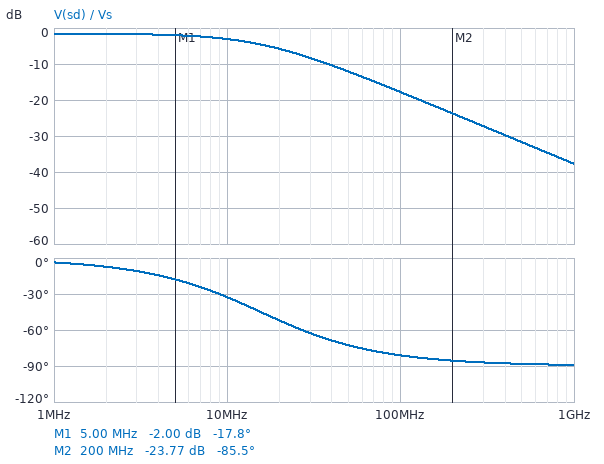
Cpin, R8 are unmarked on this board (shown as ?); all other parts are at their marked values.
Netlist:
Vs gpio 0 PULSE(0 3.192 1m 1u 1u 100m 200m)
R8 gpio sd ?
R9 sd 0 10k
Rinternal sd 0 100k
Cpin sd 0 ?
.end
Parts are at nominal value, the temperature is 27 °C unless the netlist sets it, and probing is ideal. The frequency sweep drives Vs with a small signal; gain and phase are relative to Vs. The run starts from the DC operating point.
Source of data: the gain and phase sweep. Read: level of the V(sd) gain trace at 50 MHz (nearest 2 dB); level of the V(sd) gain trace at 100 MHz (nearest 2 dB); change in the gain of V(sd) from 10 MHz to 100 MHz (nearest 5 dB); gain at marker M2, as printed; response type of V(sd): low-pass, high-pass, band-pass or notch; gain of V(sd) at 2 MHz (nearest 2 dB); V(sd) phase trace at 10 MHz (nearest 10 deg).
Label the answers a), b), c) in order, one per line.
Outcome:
a) -12 dB
b) -18 dB
c) -15 dB
d) -23.77 dB
e) low-pass
f) -2 dB
g) -30 deg
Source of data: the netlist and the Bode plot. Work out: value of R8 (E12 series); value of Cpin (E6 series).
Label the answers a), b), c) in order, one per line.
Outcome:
a) 1.8 kΩ
b) 6.8 pF
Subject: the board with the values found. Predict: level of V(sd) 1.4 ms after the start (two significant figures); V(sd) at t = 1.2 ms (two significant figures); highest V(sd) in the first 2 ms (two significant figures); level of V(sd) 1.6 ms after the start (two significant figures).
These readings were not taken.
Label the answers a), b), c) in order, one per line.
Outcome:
a) 2.7 V
b) 2.7 V
c) 2.7 V
d) 2.7 V
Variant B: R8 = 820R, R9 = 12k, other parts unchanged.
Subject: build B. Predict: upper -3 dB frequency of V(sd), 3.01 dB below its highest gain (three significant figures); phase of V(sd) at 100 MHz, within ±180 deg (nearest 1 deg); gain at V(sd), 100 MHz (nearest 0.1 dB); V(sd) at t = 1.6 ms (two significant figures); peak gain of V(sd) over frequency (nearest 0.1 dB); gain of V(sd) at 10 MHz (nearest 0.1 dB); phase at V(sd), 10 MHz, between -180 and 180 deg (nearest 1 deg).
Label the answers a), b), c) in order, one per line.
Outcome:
a) 30.7 MHz
b) -73 deg
c) -11.3 dB
d) 3.0 V
e) -0.6 dB
f) -1.1 dB
g) -18 deg
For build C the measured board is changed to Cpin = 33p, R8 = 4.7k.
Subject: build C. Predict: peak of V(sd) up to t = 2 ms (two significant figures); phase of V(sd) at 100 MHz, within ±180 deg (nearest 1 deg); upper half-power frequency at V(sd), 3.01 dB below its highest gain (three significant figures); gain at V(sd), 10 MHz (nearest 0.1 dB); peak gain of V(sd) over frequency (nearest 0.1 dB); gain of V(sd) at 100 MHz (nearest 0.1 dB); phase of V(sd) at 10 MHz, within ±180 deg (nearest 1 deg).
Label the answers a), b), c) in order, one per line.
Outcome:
a) 2.1 V
b) -89 deg
c) 1.56 MHz
d) -19.9 dB
e) -3.6 dB
f) -39.8 dB
g) -81 deg
